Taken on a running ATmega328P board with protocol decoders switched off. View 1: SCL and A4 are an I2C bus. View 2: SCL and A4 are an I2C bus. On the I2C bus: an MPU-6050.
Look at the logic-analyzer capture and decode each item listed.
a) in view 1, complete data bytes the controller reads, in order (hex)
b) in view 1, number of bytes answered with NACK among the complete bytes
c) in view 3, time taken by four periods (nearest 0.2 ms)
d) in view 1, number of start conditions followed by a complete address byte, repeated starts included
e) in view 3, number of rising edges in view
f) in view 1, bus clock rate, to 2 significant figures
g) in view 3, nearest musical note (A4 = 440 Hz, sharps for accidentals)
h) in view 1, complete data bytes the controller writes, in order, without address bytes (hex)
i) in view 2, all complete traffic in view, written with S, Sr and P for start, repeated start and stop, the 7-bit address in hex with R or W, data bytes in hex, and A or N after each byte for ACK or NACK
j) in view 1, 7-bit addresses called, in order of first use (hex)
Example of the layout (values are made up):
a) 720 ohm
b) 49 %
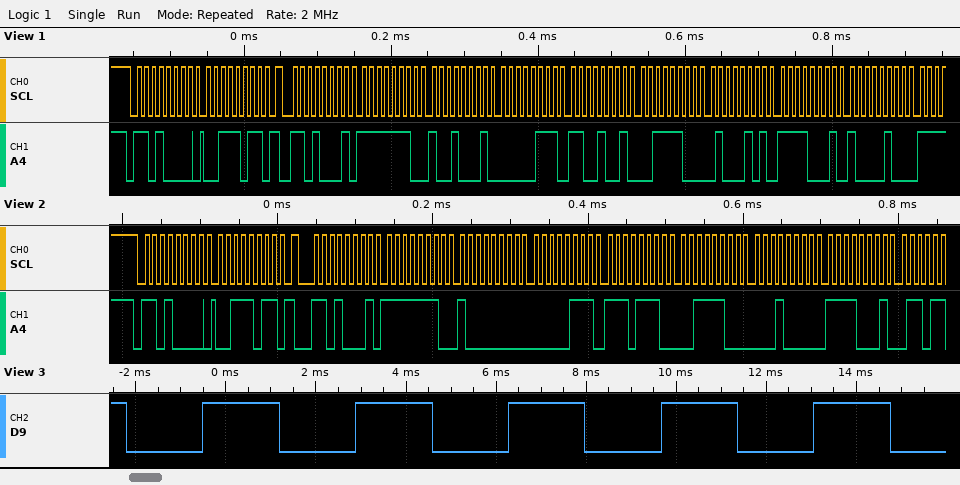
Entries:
a) FE 91 07 C9 3C 45 F1 84
b) 0
c) 13.6 ms
d) 2
e) 5
f) 100 kHz
g) D4
h) 3B
i) S 68W A 3B A Sr 68R A FE A 80 A 07 A EE A 3C A 10 A F1 A
j) 0x68
